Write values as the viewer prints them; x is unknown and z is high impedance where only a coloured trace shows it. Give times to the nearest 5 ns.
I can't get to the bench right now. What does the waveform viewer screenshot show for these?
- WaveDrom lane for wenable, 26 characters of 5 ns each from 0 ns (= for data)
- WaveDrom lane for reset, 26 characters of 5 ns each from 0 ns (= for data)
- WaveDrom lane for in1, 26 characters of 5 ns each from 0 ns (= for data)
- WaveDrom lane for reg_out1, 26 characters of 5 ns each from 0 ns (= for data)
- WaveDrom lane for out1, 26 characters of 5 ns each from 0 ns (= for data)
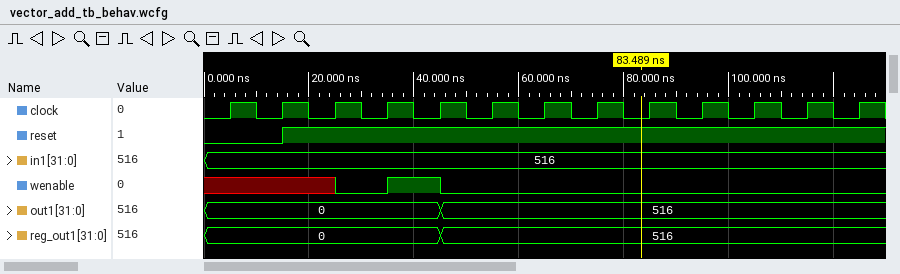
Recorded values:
{name: 'wenable', wave: 'x....0.1.0................'}
{name: 'reset', wave: '0..1......................'}
{name: 'in1', wave: '=.........................', data: '516'}
{name: 'reg_out1', wave: '=........=................', data: '0 516'}
{name: 'out1', wave: '=........=................', data: '0 516'}
